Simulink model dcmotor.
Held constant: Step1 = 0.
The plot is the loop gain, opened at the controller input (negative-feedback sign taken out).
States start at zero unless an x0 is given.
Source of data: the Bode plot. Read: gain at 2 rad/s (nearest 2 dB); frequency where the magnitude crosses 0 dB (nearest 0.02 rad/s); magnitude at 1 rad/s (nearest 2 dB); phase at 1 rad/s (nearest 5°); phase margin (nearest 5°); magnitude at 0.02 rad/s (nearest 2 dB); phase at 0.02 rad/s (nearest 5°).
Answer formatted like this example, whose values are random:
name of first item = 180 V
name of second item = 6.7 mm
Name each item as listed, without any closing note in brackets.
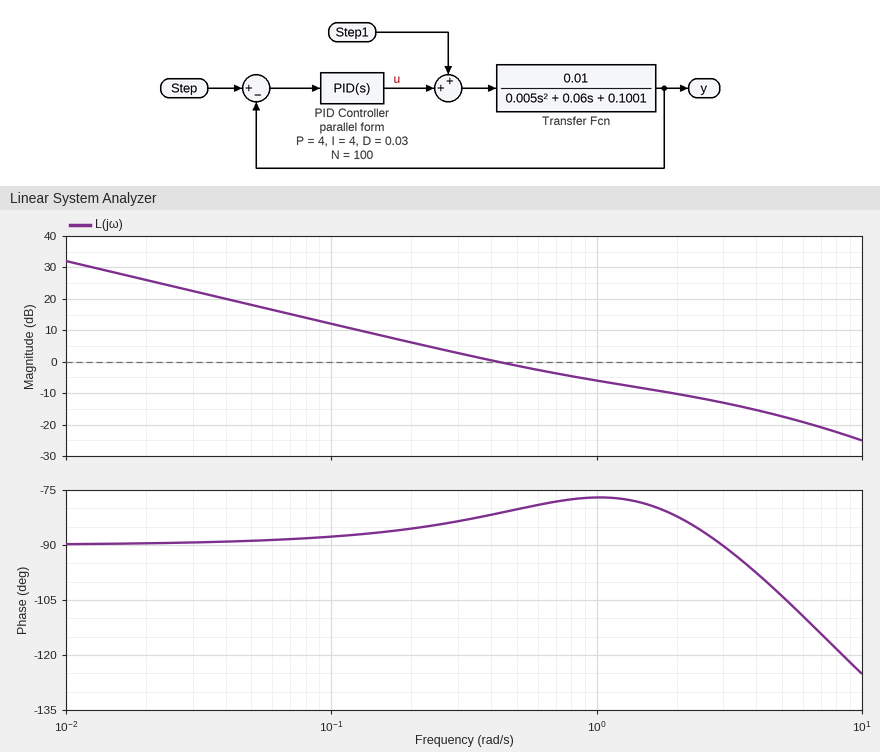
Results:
gain at 2 rad/s = -10 dB
frequency where the magnitude crosses 0 dB = 0.42 rad/s
magnitude at 1 rad/s = -6 dB
phase at 1 rad/s = -75°
phase margin = 100°
magnitude at 0.02 rad/s = 26 dB
phase at 0.02 rad/s = -90°
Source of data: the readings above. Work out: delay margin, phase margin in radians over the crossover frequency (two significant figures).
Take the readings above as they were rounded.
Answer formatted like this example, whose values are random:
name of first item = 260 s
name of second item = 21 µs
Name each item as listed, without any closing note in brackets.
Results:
delay margin, phase margin in radians over the crossover frequency = 4.2 s
